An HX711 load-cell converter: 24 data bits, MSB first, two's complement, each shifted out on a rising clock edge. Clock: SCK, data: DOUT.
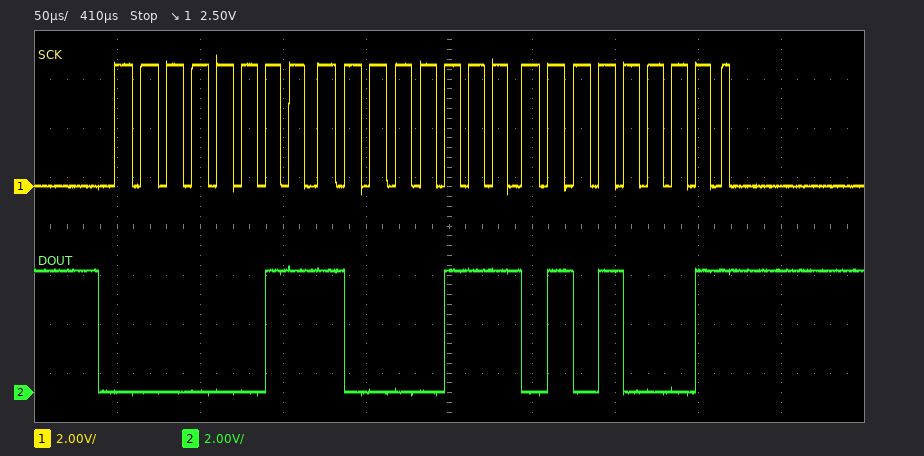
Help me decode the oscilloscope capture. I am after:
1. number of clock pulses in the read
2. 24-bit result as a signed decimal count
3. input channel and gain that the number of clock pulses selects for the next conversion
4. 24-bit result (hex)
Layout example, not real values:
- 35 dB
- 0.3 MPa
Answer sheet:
- 25
- 231249
- channel A, gain 128
- 0x038751
